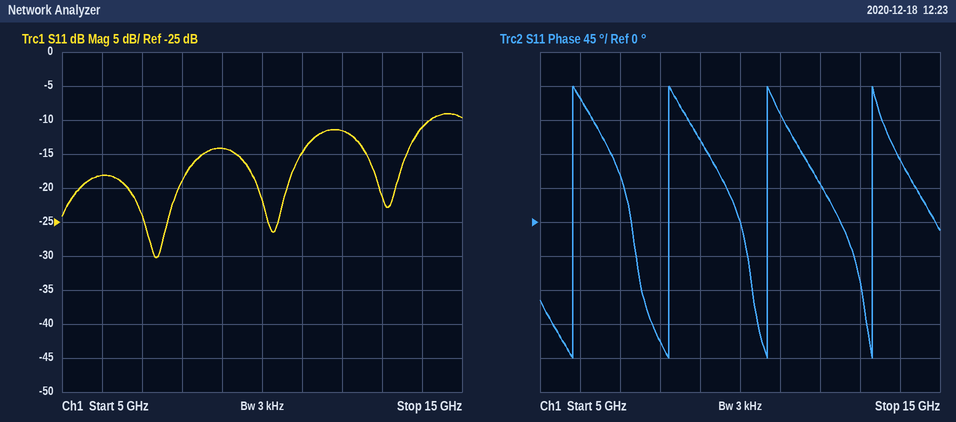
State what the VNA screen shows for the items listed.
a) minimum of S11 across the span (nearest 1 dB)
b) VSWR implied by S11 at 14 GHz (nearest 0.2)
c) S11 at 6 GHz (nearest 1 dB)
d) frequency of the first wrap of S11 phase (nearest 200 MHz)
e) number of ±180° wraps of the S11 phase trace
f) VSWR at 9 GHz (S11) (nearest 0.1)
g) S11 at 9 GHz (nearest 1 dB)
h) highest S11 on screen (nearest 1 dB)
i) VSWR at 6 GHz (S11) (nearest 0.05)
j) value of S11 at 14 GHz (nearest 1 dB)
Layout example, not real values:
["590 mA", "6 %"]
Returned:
["-30 dB", "1.8", "-18 dB", "5.8 GHz", "4", "1.5", "-14 dB", "-9 dB", "1.30", "-11 dB"]
